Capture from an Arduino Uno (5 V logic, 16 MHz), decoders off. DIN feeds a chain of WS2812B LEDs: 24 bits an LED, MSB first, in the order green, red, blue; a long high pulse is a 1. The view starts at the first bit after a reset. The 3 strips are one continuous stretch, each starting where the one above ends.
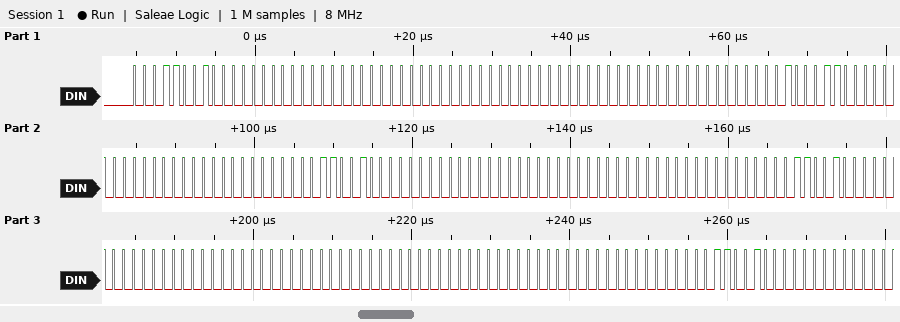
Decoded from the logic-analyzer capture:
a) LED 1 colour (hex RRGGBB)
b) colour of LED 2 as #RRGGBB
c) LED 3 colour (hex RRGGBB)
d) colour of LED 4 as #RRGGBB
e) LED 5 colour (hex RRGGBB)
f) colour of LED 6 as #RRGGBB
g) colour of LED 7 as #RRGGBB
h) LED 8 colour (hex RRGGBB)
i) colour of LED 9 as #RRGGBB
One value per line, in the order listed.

#001900
#000000
#000023
#000000
#001900
#000000
#001900
#000000
#000000
